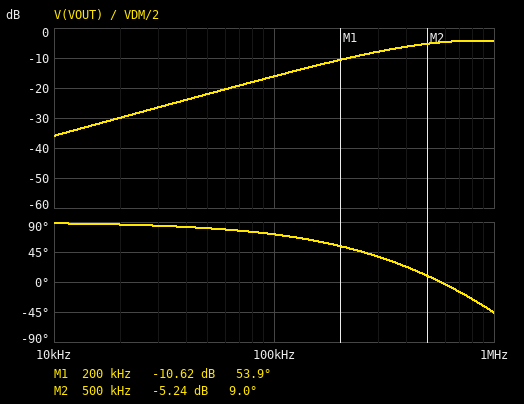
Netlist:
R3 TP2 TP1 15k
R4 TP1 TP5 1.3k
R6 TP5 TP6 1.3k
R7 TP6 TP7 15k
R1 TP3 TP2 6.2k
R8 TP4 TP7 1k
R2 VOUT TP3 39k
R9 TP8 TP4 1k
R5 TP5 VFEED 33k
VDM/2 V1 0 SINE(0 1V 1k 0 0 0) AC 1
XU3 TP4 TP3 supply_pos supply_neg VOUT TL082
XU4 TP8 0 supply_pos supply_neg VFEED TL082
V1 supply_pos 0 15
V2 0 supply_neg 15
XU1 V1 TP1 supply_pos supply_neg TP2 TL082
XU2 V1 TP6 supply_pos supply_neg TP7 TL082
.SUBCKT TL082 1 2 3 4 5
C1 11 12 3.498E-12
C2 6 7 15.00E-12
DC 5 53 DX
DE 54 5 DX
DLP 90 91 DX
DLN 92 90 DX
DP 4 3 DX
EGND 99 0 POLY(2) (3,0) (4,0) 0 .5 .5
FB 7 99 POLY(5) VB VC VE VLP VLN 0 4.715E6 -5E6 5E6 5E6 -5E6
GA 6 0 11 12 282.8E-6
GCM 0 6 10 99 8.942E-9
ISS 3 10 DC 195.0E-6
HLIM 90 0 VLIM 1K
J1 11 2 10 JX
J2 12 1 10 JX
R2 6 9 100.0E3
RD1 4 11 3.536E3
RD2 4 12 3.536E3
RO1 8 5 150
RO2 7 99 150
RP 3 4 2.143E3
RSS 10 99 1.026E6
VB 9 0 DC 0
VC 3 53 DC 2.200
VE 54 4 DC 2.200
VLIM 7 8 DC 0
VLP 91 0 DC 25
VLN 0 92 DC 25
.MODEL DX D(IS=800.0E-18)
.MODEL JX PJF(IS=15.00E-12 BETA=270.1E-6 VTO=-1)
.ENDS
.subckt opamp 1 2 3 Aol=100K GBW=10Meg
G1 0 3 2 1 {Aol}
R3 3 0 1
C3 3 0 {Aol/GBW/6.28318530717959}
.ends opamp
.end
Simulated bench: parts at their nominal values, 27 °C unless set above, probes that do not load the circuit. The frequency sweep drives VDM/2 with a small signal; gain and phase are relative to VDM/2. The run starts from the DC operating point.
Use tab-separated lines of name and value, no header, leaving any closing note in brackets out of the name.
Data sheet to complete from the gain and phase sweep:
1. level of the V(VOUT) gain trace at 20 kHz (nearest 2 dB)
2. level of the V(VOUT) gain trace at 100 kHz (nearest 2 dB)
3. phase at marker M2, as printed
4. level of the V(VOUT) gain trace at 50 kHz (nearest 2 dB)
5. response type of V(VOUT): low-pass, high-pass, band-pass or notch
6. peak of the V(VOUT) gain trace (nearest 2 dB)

level of the V(VOUT) gain trace at 20 kHz	-30 dB
level of the V(VOUT) gain trace at 100 kHz	-16 dB
phase at marker M2, as printed	9.0 deg
level of the V(VOUT) gain trace at 50 kHz	-22 dB
response type of V(VOUT): low-pass, high-pass, band-pass or notch	high-pass
peak of the V(VOUT) gain trace	-4 dB
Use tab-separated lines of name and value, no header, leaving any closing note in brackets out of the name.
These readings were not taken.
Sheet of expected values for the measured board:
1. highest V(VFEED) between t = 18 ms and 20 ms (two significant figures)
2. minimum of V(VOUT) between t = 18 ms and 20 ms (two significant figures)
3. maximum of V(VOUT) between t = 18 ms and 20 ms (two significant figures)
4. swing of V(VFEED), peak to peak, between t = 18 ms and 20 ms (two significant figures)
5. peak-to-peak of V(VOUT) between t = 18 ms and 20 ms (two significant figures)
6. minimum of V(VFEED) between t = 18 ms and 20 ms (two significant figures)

highest V(VFEED) between t = 18 ms and 20 ms	5.5 V
minimum of V(VOUT) between t = 18 ms and 20 ms	-1.5 mV
maximum of V(VOUT) between t = 18 ms and 20 ms	1.7 mV
swing of V(VFEED), peak to peak, between t = 18 ms and 20 ms	11 V
peak-to-peak of V(VOUT) between t = 18 ms and 20 ms	3.2 mV
minimum of V(VFEED) between t = 18 ms and 20 ms	-5.5 V
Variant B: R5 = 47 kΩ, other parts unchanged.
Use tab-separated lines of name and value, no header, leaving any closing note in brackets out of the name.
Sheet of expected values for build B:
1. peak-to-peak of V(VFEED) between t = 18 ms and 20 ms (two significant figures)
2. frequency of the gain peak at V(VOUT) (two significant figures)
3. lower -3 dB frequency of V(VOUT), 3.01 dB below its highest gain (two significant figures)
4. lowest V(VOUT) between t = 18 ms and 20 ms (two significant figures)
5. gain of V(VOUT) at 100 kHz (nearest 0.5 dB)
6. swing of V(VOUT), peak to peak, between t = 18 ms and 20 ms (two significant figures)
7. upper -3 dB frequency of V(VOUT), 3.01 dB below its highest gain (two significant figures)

peak-to-peak of V(VFEED) between t = 18 ms and 20 ms	15 V
frequency of the gain peak at V(VOUT)	630 kHz
lower -3 dB frequency of V(VOUT), 3.01 dB below its highest gain	260 kHz
lowest V(VOUT) between t = 18 ms and 20 ms	-2.1 mV
gain of V(VOUT) at 100 kHz	-13.5 dB
swing of V(VOUT), peak to peak, between t = 18 ms and 20 ms	4.3 mV
upper -3 dB frequency of V(VOUT), 3.01 dB below its highest gain	1.4 MHz
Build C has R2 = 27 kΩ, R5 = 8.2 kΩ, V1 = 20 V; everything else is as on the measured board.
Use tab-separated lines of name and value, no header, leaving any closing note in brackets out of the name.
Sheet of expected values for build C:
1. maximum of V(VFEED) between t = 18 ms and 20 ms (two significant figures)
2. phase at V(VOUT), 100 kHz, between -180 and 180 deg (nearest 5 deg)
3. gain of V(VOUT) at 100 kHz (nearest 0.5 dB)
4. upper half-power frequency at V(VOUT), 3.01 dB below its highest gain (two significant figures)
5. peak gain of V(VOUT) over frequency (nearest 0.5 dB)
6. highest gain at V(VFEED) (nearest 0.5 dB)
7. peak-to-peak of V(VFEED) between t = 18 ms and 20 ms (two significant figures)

maximum of V(VFEED) between t = 18 ms and 20 ms	2.2 V
phase at V(VOUT), 100 kHz, between -180 and 180 deg	80 deg
gain of V(VOUT) at 100 kHz	-24.0 dB
upper half-power frequency at V(VOUT), 3.01 dB below its highest gain	2.4 MHz
peak gain of V(VOUT) over frequency	9.5 dB
highest gain at V(VFEED)	23.5 dB
peak-to-peak of V(VFEED) between t = 18 ms and 20 ms	4.4 V
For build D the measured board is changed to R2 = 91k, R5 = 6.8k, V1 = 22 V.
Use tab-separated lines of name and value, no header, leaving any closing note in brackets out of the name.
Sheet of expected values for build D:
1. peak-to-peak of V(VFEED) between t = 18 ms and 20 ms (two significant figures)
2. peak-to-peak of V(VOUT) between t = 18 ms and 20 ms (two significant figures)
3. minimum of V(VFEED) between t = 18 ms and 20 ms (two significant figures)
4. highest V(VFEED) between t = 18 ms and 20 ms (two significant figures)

peak-to-peak of V(VFEED) between t = 18 ms and 20 ms	4.0 V
peak-to-peak of V(VOUT) between t = 18 ms and 20 ms	1.2 mV
minimum of V(VFEED) between t = 18 ms and 20 ms	-2.0 V
highest V(VFEED) between t = 18 ms and 20 ms	2.0 V
